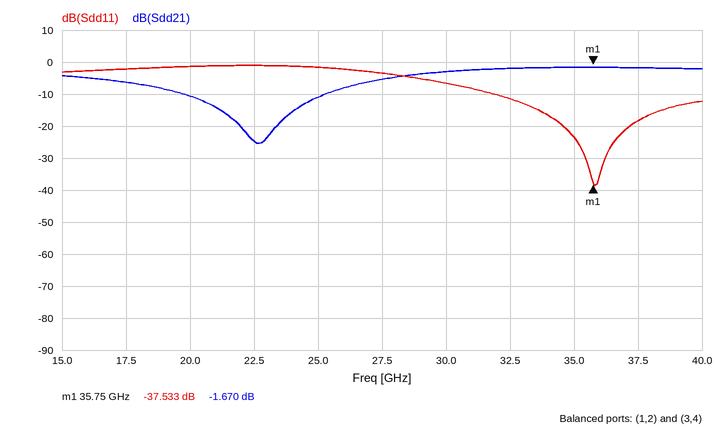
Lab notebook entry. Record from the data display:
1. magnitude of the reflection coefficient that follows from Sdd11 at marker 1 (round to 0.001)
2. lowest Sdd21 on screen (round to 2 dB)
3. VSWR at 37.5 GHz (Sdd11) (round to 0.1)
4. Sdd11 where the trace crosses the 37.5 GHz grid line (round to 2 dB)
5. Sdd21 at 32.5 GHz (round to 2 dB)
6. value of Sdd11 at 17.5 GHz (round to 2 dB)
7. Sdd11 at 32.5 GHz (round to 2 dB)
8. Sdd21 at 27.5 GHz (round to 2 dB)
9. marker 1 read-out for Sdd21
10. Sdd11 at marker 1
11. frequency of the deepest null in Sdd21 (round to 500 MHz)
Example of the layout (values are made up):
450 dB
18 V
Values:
0.013
-26 dB
1.3
-18 dB
-2 dB
-2 dB
-12 dB
-6 dB
-1.670 dB
-37.533 dB
22.5 GHz
